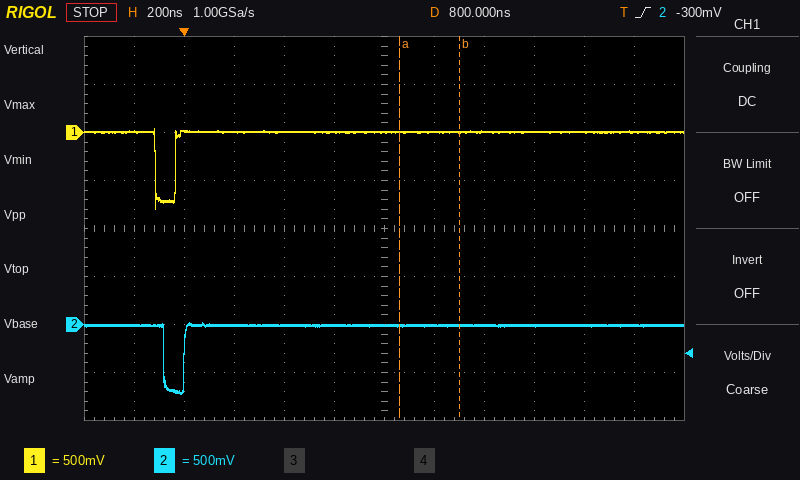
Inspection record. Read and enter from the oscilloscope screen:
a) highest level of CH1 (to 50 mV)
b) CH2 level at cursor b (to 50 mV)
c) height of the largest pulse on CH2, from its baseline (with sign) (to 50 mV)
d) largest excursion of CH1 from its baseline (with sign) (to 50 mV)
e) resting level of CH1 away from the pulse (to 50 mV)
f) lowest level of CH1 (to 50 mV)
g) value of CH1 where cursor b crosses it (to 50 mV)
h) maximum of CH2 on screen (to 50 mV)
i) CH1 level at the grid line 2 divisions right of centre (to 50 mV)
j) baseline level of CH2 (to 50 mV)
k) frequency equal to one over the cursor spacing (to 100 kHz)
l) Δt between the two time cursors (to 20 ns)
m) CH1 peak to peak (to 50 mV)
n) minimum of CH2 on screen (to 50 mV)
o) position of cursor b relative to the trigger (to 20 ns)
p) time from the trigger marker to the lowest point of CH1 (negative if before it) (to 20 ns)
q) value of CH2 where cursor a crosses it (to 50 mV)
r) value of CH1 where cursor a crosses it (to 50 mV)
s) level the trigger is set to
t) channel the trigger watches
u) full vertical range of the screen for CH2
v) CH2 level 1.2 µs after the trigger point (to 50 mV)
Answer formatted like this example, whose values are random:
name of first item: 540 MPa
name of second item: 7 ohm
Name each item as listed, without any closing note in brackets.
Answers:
highest level of CH1: 50 mV
CH2 level at cursor b: 0 mV
height of the largest pulse on CH2, from its baseline (with sign): -700 mV
largest excursion of CH1 from its baseline (with sign): -800 mV
resting level of CH1 away from the pulse: 0 mV
lowest level of CH1: -800 mV
value of CH1 where cursor b crosses it: 0 mV
maximum of CH2 on screen: 0 mV
CH1 level at the grid line 2 divisions right of centre: 0 mV
baseline level of CH2: 0 mV
frequency equal to one over the cursor spacing: 4.2 MHz
Δt between the two time cursors: 240 ns
CH1 peak to peak: 850 mV
minimum of CH2 on screen: -700 mV
position of cursor b relative to the trigger: +1.10 µs
time from the trigger marker to the lowest point of CH1 (negative if before it): -120 ns
value of CH2 where cursor a crosses it: 0 mV
value of CH1 where cursor a crosses it: 0 mV
level the trigger is set to: -300 mV
channel the trigger watches: CH2
full vertical range of the screen for CH2: 4 V
CH2 level 1.2 µs after the trigger point: 0 mV
